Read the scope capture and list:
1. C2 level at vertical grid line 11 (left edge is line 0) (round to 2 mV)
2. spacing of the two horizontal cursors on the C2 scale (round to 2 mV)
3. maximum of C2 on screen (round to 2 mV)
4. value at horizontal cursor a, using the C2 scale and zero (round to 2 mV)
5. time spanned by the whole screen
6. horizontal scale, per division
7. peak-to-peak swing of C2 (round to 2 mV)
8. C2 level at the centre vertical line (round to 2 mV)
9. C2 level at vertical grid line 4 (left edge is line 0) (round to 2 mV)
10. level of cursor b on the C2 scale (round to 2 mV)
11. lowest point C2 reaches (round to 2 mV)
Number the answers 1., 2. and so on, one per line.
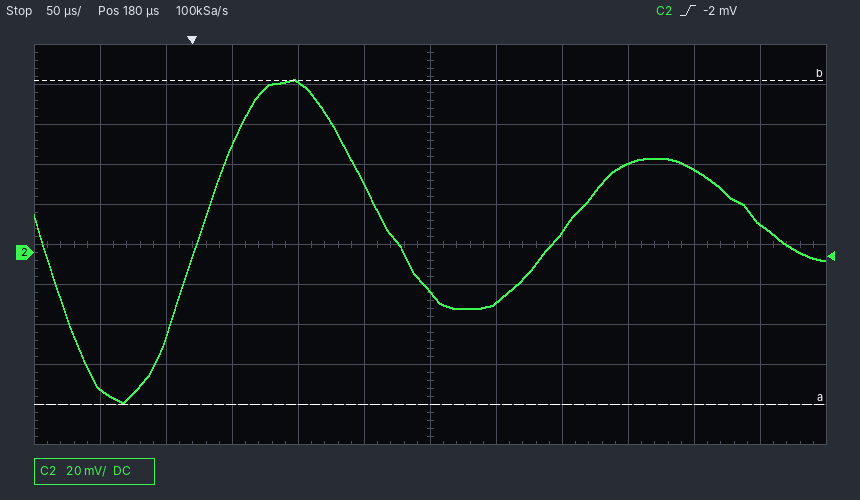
1. 14 mV
2. 162 mV
3. 86 mV
4. -76 mV
5. 600 µs
6. 50 µs
7. 162 mV
8. -20 mV
9. 86 mV
10. 86 mV
11. -76 mV
